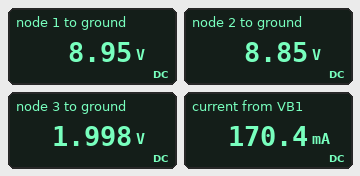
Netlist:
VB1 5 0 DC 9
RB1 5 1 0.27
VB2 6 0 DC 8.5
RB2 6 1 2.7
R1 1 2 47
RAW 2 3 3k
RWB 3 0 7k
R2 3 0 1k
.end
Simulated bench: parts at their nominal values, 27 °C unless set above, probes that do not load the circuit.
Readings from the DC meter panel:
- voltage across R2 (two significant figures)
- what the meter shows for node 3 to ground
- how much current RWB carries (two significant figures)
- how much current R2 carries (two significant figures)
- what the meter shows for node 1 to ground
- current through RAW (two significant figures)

2.0 V
1.998 V
290 µA
2.0 mA
8.95 V
2.3 mA
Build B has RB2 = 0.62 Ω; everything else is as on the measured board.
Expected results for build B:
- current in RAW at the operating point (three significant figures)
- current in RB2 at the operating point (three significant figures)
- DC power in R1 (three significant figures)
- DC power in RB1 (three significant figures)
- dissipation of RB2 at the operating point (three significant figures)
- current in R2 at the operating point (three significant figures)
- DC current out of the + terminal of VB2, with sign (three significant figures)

2.26 mA
561 mA
239 µW
85.7 mW
195 mW
1.97 mA
-561 mA
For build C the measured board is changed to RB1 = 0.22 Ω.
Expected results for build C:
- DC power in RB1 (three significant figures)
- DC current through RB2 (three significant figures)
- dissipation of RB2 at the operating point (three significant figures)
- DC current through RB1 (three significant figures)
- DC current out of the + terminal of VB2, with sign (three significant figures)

6.61 mW
171 mA
79.0 mW
173 mA
-171 mA
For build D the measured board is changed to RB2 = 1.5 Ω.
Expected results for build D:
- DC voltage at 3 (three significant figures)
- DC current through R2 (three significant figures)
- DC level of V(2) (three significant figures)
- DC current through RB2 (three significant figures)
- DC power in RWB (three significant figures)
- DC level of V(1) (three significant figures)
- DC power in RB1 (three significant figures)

1.99 V
1.99 mA
8.82 V
282 mA
566 µW
8.92 V
21.8 mW
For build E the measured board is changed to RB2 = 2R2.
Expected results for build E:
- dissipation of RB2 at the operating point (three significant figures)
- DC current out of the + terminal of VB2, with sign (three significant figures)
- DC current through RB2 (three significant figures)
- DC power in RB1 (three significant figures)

89.9 mW
-202 mA
202 mA
11.3 mW
